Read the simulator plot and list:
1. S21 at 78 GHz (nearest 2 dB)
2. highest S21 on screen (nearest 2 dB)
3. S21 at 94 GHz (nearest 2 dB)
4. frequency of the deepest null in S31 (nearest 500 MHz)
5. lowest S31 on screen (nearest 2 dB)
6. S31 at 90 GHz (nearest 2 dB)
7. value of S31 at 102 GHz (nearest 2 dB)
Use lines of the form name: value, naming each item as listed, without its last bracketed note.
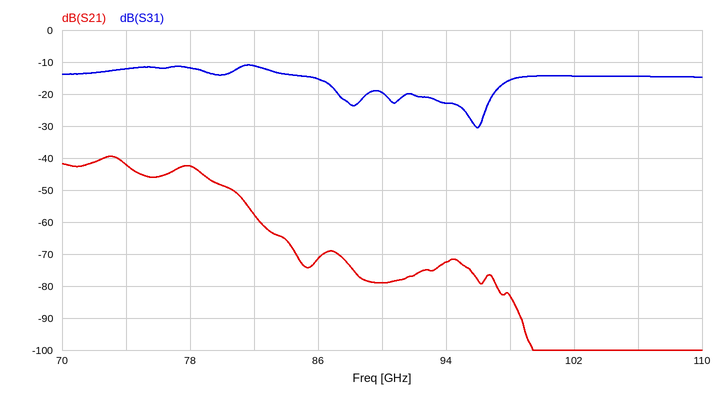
S21 at 78 GHz: -42 dB
highest S21 on screen: -40 dB
S21 at 94 GHz: -72 dB
frequency of the deepest null in S31: 96.0 GHz
lowest S31 on screen: -30 dB
S31 at 90 GHz: -20 dB
value of S31 at 102 GHz: -14 dB
